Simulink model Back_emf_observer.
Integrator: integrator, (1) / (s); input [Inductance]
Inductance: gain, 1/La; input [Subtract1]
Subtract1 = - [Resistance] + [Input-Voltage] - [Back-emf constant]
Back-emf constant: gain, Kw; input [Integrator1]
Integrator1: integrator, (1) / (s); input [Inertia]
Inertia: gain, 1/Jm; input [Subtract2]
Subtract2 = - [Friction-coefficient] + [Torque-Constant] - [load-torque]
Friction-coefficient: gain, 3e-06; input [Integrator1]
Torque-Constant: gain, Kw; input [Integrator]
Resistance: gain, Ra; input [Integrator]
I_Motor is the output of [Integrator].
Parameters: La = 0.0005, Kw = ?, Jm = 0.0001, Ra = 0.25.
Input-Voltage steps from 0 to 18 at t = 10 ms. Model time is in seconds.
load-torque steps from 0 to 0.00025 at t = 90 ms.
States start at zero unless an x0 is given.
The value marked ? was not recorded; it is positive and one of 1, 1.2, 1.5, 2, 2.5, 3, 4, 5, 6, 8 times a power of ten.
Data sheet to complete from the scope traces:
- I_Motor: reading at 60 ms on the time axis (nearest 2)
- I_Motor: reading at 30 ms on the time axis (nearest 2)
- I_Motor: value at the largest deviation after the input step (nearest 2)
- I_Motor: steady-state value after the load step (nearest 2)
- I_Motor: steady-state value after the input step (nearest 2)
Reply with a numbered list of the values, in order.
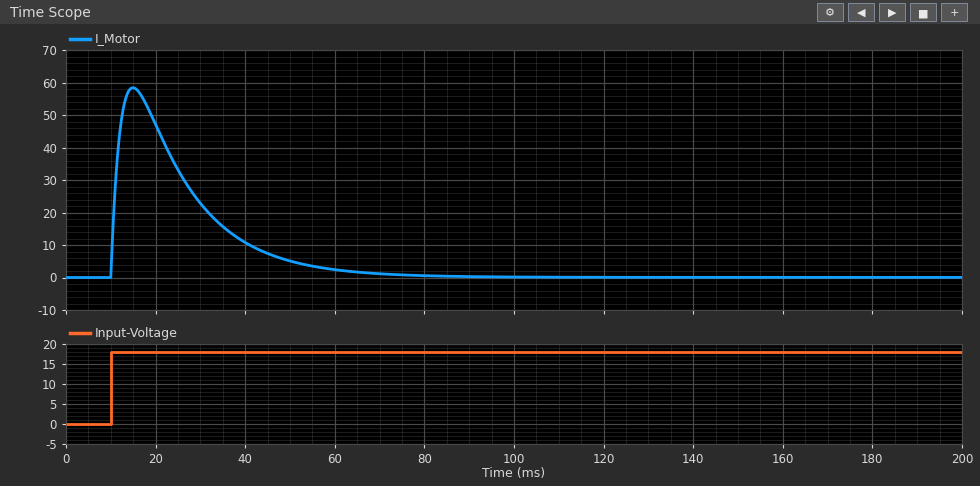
1. 2
2. 22
3. 58
4. 0
5. 0
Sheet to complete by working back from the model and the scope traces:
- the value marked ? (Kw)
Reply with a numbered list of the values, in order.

1. 0.04
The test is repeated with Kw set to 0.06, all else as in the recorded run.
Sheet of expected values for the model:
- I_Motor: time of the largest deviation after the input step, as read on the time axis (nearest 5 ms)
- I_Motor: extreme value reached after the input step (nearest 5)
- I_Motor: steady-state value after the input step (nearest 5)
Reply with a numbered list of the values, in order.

1. 15 ms
2. 50
3. 0
